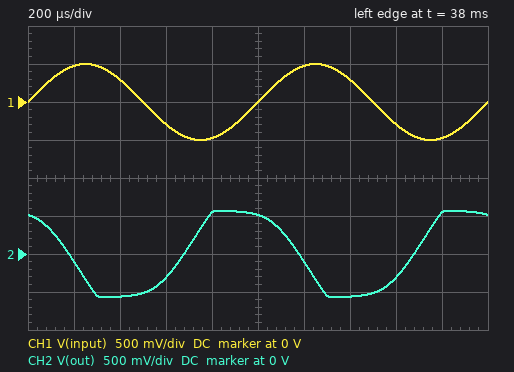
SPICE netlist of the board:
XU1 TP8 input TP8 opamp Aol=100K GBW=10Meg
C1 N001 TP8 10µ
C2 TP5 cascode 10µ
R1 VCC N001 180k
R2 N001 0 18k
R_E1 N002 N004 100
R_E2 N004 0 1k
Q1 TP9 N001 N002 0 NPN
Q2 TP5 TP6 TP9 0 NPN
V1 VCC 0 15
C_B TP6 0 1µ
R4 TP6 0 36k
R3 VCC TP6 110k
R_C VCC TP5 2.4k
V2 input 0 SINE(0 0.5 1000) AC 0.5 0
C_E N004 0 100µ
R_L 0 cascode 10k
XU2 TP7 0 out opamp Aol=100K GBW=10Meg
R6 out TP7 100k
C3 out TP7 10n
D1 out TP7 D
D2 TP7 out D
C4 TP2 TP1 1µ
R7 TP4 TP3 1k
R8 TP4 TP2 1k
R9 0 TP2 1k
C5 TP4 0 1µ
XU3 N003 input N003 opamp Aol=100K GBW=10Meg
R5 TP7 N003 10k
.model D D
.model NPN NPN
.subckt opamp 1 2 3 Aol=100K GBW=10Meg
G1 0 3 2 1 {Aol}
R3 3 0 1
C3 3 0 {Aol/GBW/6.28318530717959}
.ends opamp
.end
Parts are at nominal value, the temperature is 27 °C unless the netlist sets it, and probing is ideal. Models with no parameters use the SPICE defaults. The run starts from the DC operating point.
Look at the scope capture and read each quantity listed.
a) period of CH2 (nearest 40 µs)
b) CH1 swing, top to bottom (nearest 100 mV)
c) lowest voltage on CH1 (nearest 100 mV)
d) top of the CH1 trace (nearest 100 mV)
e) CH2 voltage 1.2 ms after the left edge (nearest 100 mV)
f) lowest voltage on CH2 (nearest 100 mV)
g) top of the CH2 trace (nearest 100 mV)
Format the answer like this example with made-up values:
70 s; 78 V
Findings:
1.00 ms; 1.0 V; -500 mV; 500 mV; -100 mV; -600 mV; 600 mV
